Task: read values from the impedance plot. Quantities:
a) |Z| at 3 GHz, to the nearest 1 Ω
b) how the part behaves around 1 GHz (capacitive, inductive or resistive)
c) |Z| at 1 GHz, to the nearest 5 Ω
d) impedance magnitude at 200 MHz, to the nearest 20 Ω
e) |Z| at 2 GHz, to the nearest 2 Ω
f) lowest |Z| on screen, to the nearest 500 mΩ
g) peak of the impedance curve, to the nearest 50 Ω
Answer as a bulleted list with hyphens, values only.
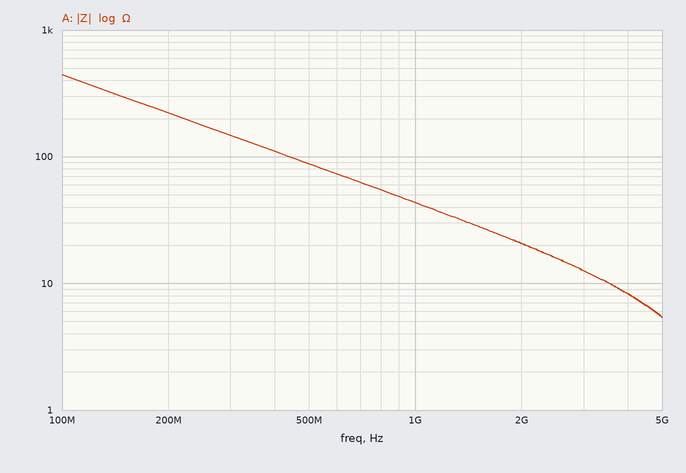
- 13 Ω
- capacitive
- 45 Ω
- 220 Ω
- 20 Ω
- 5.5 Ω
- 450 Ω
